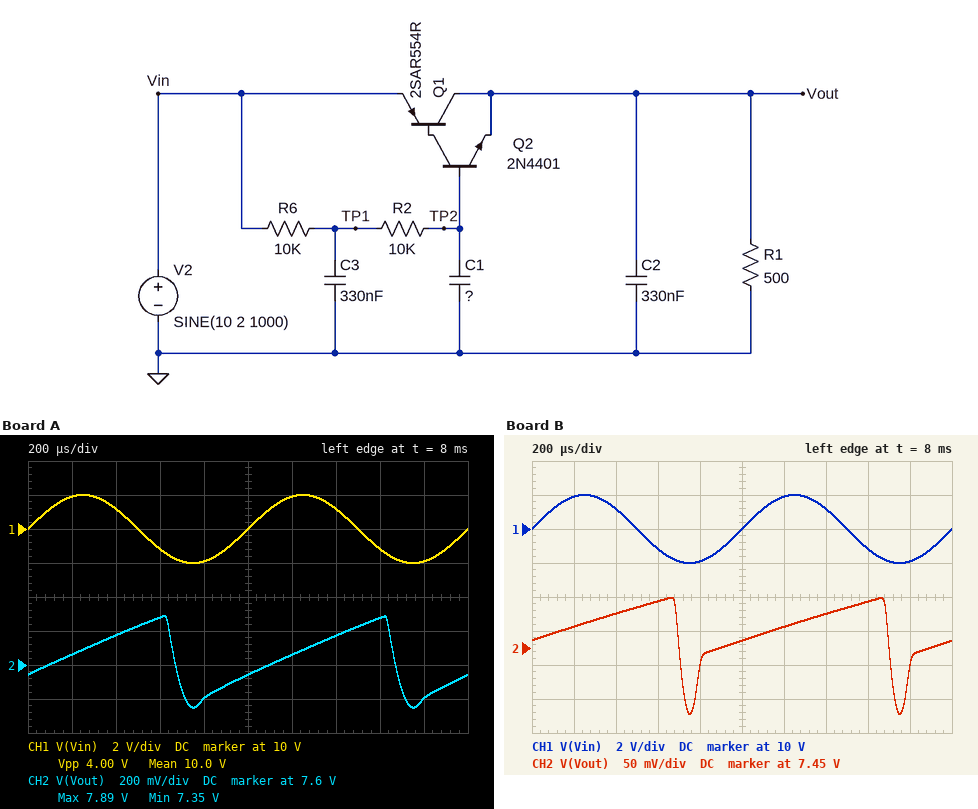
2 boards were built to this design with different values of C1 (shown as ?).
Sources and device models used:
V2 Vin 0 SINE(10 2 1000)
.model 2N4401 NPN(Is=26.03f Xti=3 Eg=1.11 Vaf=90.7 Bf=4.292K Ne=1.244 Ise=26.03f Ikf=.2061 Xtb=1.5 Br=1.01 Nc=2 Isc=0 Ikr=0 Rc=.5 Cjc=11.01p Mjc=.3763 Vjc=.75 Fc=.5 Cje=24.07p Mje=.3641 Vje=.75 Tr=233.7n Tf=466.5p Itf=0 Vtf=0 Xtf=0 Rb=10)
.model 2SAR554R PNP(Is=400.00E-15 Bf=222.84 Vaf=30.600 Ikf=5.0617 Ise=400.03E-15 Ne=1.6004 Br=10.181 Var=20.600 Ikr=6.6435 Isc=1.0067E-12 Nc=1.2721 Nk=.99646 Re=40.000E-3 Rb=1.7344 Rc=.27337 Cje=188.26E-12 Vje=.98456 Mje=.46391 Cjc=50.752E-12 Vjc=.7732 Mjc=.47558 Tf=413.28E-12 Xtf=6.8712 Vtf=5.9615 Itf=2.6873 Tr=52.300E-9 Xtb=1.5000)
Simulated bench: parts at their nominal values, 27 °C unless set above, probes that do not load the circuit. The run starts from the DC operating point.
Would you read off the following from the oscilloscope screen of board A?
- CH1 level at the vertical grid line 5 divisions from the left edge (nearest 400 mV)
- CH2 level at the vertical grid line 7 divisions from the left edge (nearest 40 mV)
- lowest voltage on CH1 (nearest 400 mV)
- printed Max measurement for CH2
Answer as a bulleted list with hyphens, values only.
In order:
- 10.0 V
- 7.76 V
- 8.0 V
- 7.89 V
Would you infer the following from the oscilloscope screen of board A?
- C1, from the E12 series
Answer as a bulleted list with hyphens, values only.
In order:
- 150 nF
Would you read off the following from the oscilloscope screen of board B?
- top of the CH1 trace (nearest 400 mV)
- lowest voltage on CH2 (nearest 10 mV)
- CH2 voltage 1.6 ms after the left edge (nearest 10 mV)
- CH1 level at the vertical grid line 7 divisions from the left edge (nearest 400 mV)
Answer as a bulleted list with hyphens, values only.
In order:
- 12.0 V
- 7.35 V
- 7.52 V
- 11.2 V
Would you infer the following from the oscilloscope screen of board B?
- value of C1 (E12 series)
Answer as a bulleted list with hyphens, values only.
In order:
- 1 µF
